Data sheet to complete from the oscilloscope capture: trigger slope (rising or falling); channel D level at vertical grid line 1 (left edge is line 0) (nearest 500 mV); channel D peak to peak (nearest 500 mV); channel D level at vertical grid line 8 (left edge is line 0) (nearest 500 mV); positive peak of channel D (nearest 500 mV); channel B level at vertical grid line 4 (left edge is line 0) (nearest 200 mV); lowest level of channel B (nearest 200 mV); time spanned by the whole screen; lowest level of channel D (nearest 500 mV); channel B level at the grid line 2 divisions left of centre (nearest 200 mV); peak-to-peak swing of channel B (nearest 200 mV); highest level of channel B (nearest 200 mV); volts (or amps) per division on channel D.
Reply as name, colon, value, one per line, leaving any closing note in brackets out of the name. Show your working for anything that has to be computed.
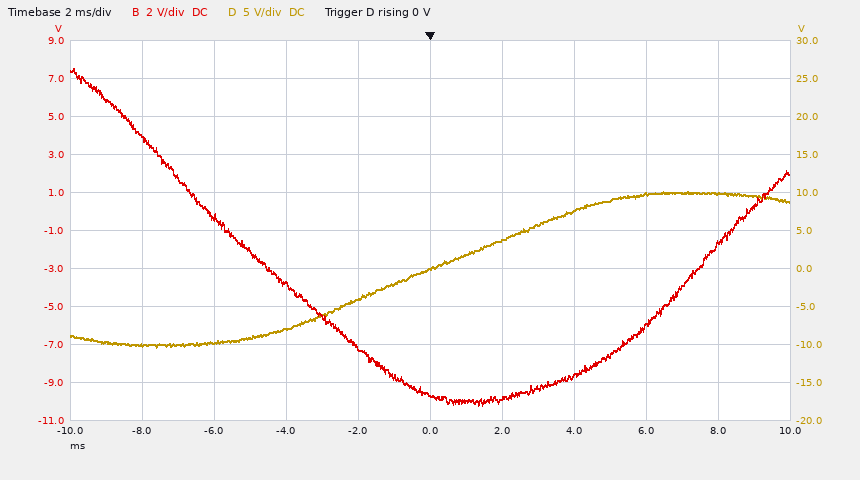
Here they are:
trigger slope: rising
channel D level at vertical grid line 1 (left edge is line 0): -10.0 V
channel D peak to peak: 10.0 V − (-10.5 V) = 20.5 V
channel D level at vertical grid line 8 (left edge is line 0): 10.0 V
positive peak of channel D: 10.0 V
channel B level at vertical grid line 4 (left edge is line 0): -7.2 V
lowest level of channel B: -10.2 V
time spanned by the whole screen: 20 ms
lowest level of channel D: -10.5 V
channel B level at the grid line 2 divisions left of centre: -3.8 V
peak-to-peak swing of channel B: 7.6 V − (-10.2 V) = 17.8 V
highest level of channel B: 7.6 V
volts (or amps) per division on channel D: 5 V
